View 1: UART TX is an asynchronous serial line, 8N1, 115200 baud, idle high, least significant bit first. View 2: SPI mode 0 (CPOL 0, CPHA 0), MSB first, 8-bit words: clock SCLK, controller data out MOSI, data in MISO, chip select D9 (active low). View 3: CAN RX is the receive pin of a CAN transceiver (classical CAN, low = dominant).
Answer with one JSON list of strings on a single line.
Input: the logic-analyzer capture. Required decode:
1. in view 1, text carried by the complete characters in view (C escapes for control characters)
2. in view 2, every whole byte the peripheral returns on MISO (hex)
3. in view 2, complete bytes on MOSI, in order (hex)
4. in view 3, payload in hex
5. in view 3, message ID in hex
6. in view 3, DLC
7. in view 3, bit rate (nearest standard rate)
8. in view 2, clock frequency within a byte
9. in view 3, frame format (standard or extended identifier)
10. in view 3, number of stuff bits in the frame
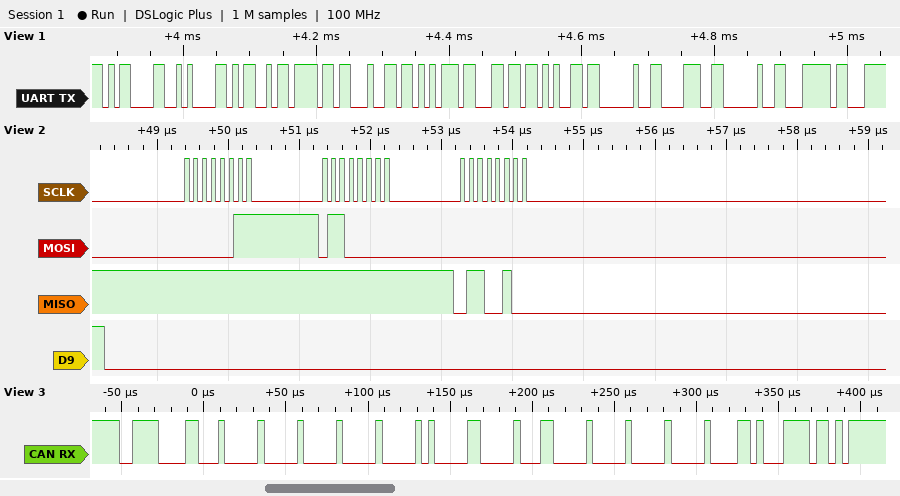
["\"\\r\\nModule 8 |\"", "FF FF 64", "03 60 00", "00 00 01 04 03 00 00 00", "0x3C3", "8", "250 kbit/s", "8 MHz", "standard", "11"]
